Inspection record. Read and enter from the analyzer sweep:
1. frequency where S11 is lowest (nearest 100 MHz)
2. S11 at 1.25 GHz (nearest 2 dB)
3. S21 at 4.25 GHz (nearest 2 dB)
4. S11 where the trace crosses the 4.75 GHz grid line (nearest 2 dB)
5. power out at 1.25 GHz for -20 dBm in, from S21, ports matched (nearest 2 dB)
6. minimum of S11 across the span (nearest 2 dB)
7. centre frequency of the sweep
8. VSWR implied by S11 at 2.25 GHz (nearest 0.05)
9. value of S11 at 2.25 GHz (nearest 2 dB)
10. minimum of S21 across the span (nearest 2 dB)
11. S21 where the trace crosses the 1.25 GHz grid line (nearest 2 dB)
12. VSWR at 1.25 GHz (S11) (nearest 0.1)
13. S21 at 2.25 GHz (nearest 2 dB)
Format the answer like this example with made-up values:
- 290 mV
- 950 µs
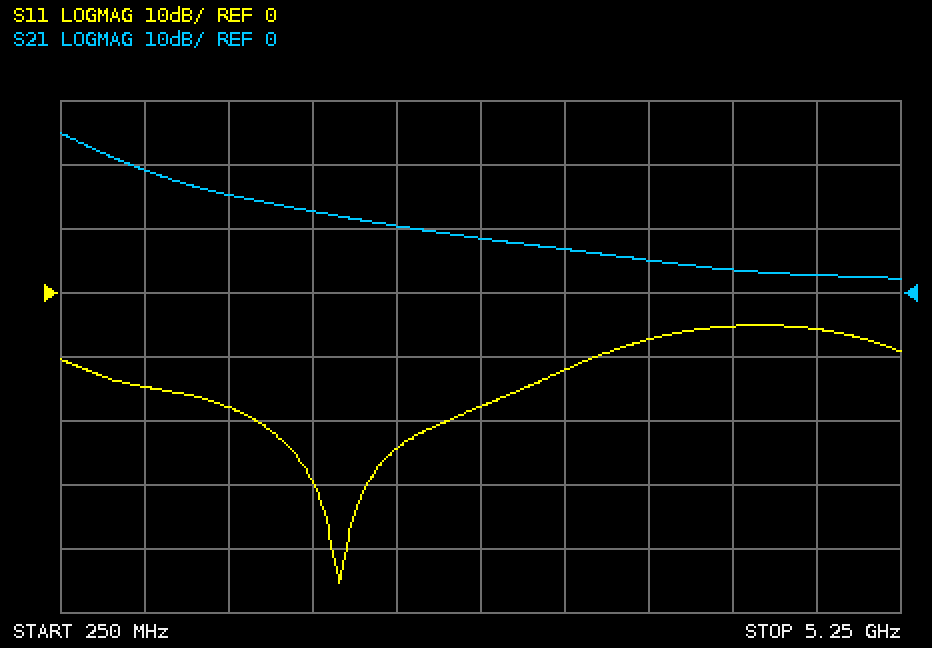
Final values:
- 1.9 GHz
- -18 dB
- 4 dB
- -6 dB
- -4 dBm
- -46 dB
- 2.75 GHz
- 1.15
- -24 dB
- 2 dB
- 16 dB
- 1.3
- 10 dB
